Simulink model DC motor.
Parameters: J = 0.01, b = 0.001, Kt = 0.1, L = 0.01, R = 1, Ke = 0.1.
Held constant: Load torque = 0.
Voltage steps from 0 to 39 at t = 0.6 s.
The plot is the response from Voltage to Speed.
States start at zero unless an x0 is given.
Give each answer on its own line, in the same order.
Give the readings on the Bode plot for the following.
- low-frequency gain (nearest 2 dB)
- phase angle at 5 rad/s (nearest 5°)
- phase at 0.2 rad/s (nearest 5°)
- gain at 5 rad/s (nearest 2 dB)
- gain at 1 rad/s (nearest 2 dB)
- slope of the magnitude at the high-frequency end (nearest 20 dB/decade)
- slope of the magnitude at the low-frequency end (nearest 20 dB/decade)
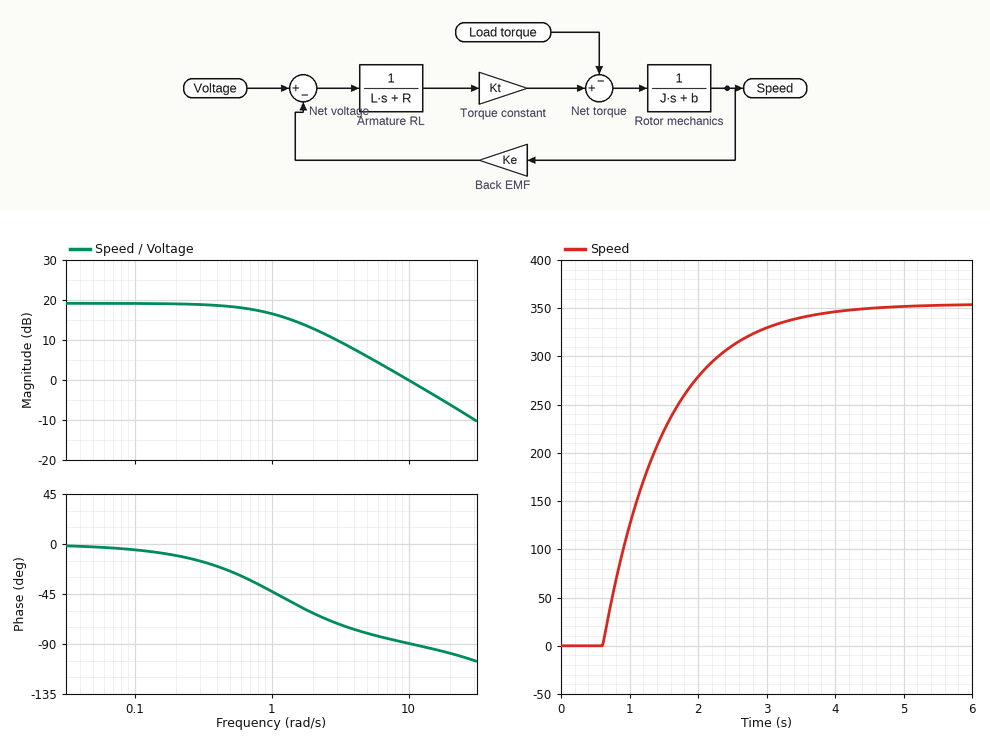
20 dB
-80°
-10°
6 dB
16 dB
-20 dB/decade
0 dB/decade
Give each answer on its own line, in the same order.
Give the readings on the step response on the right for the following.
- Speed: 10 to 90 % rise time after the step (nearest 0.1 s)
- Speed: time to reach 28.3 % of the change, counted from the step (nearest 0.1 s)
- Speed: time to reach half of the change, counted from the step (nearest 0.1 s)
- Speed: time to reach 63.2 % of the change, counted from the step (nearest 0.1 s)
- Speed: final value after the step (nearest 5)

2.0 s
0.3 s
0.6 s
0.9 s
355
